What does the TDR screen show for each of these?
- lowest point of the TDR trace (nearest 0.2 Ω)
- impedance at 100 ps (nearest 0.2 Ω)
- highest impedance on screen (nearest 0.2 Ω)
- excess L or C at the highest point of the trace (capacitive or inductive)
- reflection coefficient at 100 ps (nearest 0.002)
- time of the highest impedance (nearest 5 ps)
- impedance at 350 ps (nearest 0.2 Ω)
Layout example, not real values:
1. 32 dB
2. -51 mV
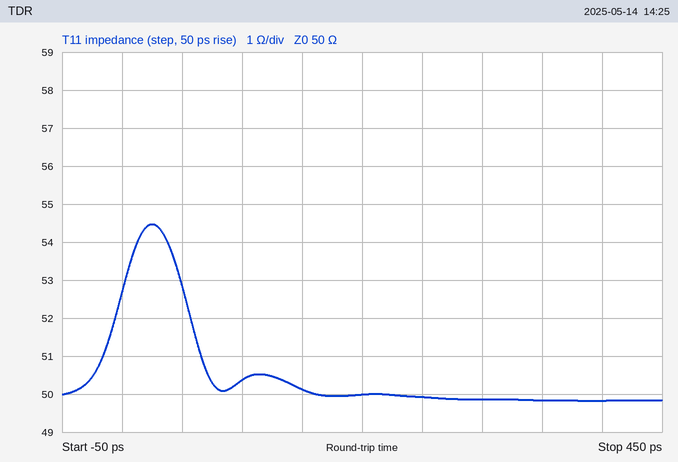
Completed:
1. 49.8 Ω
2. 50.4 Ω
3. 54.4 Ω
4. inductive
5. +0.004
6. 25 ps
7. 49.8 Ω
